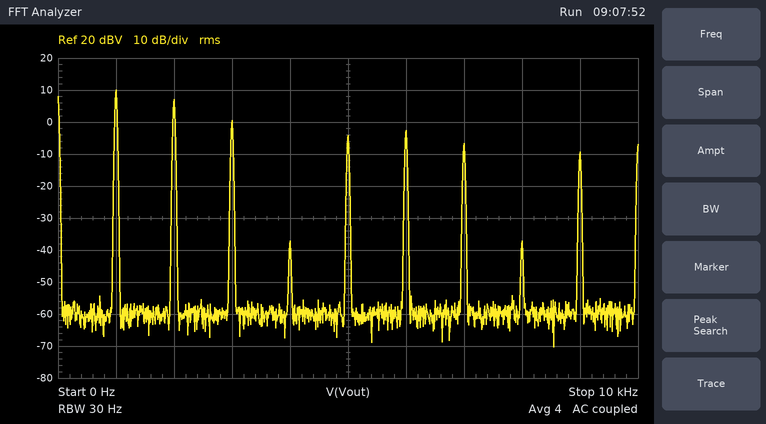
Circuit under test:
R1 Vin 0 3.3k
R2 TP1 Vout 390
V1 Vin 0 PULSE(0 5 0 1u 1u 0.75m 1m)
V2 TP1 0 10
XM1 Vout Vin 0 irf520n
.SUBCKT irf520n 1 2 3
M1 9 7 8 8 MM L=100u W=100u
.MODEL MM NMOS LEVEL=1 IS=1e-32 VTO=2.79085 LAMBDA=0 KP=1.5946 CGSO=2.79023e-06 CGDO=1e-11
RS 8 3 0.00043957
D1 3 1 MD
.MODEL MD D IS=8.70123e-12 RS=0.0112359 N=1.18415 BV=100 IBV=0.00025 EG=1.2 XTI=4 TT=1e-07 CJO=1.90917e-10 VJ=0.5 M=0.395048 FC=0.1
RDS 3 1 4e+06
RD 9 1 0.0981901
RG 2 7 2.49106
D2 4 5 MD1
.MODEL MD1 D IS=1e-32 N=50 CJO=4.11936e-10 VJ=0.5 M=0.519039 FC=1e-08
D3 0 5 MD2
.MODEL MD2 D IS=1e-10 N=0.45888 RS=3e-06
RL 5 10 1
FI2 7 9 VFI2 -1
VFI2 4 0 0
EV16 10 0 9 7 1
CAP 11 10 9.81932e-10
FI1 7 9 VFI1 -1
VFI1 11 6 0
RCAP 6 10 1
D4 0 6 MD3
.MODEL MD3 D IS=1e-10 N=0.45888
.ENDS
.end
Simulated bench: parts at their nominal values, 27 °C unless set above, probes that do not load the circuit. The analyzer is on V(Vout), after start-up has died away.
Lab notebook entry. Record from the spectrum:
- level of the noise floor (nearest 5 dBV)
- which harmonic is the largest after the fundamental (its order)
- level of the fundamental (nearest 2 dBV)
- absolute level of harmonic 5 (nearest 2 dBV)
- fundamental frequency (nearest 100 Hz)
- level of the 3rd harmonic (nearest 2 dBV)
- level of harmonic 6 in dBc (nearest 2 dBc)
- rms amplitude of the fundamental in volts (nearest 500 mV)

-60 dBV
2
10 dBV
-4 dBV
1.0 kHz
0 dBV
-12 dBc
3.0 V
